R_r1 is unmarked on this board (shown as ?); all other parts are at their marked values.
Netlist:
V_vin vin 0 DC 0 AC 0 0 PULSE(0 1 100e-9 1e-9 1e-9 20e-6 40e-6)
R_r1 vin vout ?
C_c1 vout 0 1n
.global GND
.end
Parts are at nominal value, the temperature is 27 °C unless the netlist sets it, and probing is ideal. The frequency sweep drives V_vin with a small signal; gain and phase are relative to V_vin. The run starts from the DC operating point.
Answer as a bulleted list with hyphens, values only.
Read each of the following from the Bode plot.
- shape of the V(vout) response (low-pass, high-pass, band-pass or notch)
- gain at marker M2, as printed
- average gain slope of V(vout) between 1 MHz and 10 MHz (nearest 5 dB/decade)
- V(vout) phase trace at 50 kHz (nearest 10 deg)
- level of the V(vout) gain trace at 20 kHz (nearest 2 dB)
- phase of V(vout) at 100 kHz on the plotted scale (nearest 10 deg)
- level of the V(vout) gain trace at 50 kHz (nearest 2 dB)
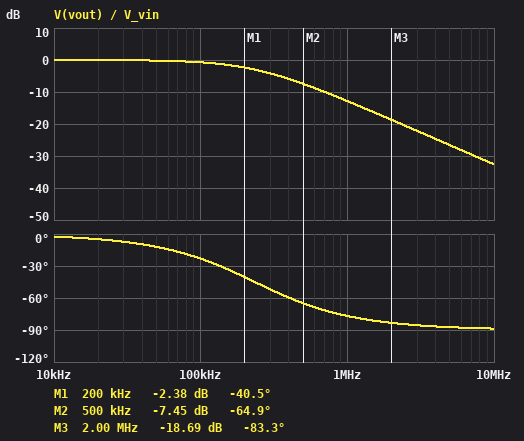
- low-pass
- -7.45 dB
- -20 dB/decade
- -10 deg
- 0 dB
- -20 deg
- 0 dB
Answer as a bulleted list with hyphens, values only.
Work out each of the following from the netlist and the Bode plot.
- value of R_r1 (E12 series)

- 680 Ω
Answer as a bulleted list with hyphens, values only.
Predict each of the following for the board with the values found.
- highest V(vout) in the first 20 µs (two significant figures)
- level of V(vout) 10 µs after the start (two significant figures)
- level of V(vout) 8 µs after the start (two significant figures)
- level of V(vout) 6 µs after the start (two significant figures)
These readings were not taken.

- 1.0 V
- 1.0 V
- 1.0 V
- 1.0 V
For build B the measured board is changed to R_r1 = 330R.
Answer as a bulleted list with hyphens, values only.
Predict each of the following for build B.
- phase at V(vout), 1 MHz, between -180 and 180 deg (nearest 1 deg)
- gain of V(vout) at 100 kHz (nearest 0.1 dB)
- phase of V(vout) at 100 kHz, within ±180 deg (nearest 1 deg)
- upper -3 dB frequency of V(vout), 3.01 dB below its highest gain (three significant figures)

- -64 deg
- -0.2 dB
- -12 deg
- 482 kHz
